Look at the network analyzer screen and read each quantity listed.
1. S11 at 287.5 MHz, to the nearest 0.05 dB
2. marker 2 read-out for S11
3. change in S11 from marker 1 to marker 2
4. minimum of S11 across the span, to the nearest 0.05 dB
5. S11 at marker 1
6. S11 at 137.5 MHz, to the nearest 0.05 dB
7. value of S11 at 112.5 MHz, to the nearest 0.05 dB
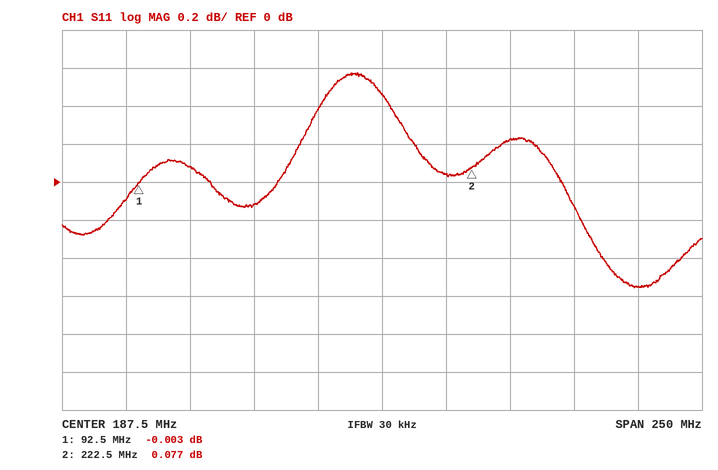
-0.55 dB
0.077 dB
0.080 dB
-0.55 dB
-0.003 dB
-0.10 dB
0.10 dB
